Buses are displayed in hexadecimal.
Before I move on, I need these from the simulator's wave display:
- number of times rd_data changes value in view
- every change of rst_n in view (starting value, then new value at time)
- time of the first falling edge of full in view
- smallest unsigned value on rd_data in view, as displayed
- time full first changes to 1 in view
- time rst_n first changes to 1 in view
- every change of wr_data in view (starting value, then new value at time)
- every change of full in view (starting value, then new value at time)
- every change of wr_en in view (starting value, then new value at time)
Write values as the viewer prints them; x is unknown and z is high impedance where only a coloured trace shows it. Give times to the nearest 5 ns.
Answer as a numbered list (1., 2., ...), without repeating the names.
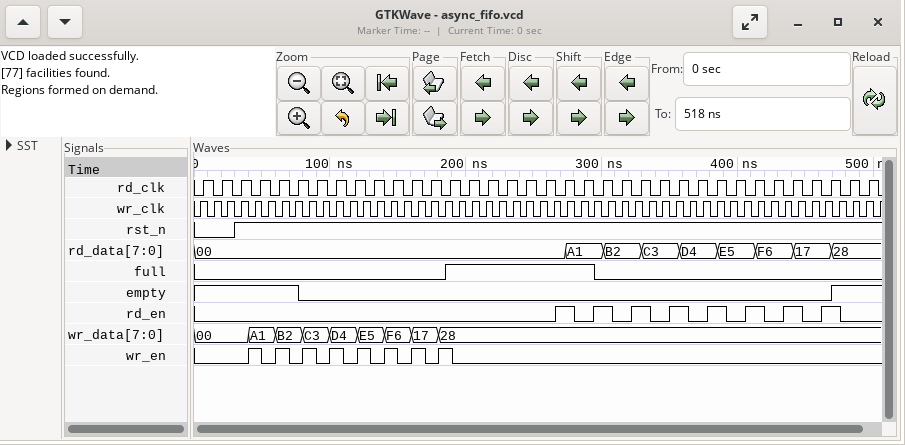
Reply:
1. 8
2. 0, 1 at 30 ns
3. 295 ns
4. 00
5. 185 ns
6. 30 ns
7. 00, A1 at 40 ns, B2 at 60 ns, C3 at 80 ns, D4 at 100 ns, E5 at 120 ns, F6 at 140 ns, 17 at 160 ns, 28 at 180 ns
8. 0, 1 at 185 ns, 0 at 295 ns
9. 0, 1 at 40 ns, 0 at 50 ns, 1 at 60 ns, 0 at 70 ns, 1 at 80 ns, 0 at 90 ns, 1 at 100 ns, 0 at 110 ns, 1 at 120 ns, 0 at 130 ns, 1 at 140 ns, 0 at 150 ns, 1 at 160 ns, 0 at 170 ns, 1 at 180 ns, 0 at 190 ns
